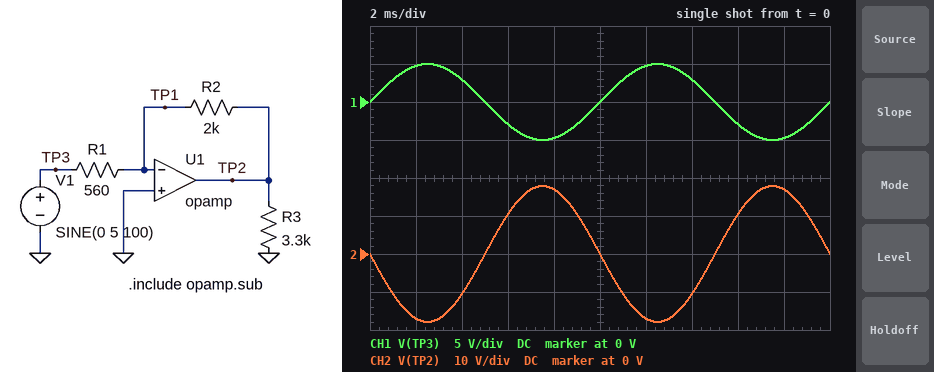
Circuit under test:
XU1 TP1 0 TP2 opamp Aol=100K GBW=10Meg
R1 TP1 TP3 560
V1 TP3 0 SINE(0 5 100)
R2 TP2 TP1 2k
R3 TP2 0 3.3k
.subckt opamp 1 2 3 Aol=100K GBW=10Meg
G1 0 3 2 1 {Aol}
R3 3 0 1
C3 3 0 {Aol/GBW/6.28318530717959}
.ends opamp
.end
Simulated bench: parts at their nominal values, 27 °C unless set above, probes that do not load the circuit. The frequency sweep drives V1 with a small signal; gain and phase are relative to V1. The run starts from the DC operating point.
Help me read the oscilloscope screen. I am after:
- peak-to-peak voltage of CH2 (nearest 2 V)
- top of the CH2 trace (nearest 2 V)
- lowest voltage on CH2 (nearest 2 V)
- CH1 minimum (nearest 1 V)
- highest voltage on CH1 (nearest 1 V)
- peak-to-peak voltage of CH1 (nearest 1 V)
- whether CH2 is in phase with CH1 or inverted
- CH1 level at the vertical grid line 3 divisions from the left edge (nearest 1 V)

36 V
18 V
-18 V
-5 V
5 V
10 V
inverted
-3 V
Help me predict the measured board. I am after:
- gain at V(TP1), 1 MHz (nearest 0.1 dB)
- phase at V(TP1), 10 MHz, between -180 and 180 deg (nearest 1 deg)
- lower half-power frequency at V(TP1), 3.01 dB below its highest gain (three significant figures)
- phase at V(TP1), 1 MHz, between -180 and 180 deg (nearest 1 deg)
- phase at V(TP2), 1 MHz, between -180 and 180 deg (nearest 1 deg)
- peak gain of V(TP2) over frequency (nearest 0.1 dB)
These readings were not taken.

-9.8 dB
12 deg
2.19 MHz
65 deg
155 deg
11.1 dB
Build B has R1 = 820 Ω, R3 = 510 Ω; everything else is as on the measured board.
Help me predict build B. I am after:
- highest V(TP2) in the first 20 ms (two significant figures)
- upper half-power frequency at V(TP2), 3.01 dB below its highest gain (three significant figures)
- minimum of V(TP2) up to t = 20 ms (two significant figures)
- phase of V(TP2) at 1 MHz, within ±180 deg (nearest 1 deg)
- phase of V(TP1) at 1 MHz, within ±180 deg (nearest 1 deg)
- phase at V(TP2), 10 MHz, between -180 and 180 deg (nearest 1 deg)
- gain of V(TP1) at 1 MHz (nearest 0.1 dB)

12 V
2.91 MHz
-12 V
161 deg
71 deg
106 deg
-12.7 dB
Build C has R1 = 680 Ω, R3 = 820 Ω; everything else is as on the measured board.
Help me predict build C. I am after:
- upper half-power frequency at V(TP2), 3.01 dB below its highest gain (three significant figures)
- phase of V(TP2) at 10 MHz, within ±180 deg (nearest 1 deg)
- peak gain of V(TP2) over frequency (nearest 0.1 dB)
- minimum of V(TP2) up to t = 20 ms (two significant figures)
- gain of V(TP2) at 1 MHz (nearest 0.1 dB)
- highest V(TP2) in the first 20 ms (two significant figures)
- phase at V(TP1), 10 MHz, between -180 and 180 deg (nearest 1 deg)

2.54 MHz
104 deg
9.4 dB
-15 V
8.7 dB
15 V
14 deg
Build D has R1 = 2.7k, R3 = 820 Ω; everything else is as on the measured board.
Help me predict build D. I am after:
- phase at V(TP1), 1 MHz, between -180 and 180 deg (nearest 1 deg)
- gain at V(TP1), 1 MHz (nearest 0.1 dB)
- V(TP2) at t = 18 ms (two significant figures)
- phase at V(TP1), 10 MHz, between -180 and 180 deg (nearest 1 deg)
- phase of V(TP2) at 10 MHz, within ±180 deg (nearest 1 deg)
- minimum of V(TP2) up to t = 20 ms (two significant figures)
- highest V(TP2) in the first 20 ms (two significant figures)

80 deg
-22.7 dB
3.5 V
30 deg
120 deg
-3.7 V
3.7 V
